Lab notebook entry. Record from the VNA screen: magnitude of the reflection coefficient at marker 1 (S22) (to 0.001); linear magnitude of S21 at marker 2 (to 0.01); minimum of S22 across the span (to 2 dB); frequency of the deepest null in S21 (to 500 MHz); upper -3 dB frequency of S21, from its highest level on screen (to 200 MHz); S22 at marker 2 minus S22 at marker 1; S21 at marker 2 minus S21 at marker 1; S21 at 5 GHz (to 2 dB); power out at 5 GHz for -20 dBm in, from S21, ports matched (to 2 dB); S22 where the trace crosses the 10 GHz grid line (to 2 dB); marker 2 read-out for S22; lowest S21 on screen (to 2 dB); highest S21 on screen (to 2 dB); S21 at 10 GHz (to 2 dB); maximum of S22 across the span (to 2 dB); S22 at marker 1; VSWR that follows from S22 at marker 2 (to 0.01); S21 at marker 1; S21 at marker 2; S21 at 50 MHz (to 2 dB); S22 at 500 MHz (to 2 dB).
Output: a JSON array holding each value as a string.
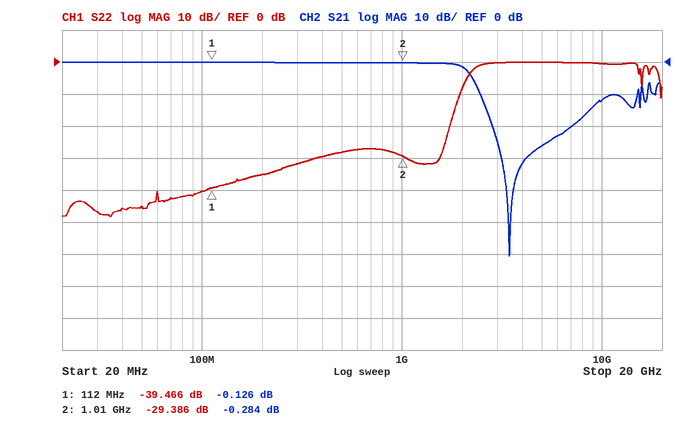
["0.011", "0.97", "-48 dB", "3.5 GHz", "2.2 GHz", "10.080 dB", "-0.158 dB", "-26 dB", "-46 dBm", "0 dB", "-29.386 dB", "-60 dB", "0 dB", "-12 dB", "0 dB", "-39.466 dB", "1.07", "-0.126 dB", "-0.284 dB", "0 dB", "-28 dB"]
